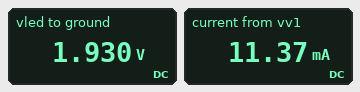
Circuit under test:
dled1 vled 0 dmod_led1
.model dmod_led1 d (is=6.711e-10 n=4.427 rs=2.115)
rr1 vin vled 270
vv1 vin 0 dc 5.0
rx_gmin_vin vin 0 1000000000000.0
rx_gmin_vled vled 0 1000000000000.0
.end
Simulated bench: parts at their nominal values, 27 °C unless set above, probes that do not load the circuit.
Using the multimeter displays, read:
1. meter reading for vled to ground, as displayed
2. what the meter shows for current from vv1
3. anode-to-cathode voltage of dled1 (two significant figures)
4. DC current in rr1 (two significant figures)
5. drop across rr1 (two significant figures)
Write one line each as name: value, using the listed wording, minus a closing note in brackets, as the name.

meter reading for vled to ground, as displayed: 1.930 V
what the meter shows for current from vv1: 11.37 mA
anode-to-cathode voltage of dled1: 1.9 V
DC current in rr1: 11 mA
drop across rr1: 3.1 V
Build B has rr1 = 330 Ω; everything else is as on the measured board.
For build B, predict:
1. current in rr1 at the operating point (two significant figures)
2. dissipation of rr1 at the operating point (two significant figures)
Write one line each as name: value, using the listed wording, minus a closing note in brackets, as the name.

current in rr1 at the operating point: 9.4 mA
dissipation of rr1 at the operating point: 29 mW
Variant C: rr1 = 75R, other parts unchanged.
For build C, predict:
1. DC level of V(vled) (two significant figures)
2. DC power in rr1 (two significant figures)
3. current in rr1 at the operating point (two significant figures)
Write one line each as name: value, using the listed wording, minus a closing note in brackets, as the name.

DC level of V(vled): 2.1 V
DC power in rr1: 110 mW
current in rr1 at the operating point: 38 mA
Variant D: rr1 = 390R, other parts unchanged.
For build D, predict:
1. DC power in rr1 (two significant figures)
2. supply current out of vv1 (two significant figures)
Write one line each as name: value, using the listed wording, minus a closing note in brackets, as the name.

DC power in rr1: 25 mW
supply current out of vv1: 8.0 mA
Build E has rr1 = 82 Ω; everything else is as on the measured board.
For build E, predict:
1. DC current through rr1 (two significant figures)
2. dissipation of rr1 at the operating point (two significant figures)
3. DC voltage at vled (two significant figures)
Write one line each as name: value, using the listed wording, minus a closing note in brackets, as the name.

DC current through rr1: 35 mA
dissipation of rr1 at the operating point: 100 mW
DC voltage at vled: 2.1 V
